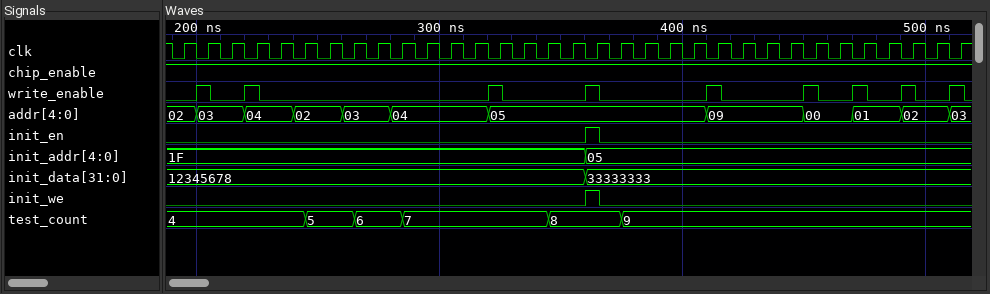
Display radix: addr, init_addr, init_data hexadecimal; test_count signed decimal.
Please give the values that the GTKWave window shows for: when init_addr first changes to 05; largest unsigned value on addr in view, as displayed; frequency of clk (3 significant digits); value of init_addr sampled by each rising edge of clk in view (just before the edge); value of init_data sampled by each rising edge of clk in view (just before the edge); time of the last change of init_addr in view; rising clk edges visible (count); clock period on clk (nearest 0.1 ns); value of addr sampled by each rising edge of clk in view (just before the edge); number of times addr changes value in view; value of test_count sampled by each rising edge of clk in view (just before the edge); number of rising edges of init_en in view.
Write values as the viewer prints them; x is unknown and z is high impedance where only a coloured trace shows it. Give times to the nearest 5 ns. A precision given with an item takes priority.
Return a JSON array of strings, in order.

["360 ns", "09", "100 MHz", "1F, 1F, 1F, 1F, 1F, 1F, 1F, 1F, 1F, 1F, 1F, 1F, 1F, 1F, 1F, 1F, 1F, 05, 05, 05, 05, 05, 05, 05, 05, 05, 05, 05, 05, 05, 05, 05, 05", "12345678, 12345678, 12345678, 12345678, 12345678, 12345678, 12345678, 12345678, 12345678, 12345678, 12345678, 12345678, 12345678, 12345678, 12345678, 12345678, 12345678, 33333333, 33333333, 33333333, 33333333, 33333333, 33333333, 33333333, 33333333, 33333333, 33333333, 33333333, 33333333, 33333333, 33333333, 33333333, 33333333", "360 ns", "33", "10 ns", "02, 03, 03, 04, 04, 02, 02, 03, 03, 04, 04, 04, 04, 05, 05, 05, 05, 05, 05, 05, 05, 05, 09, 09, 09, 09, 00, 00, 01, 01, 02, 02, 03", "11", "4, 4, 4, 4, 4, 4, 5, 5, 6, 6, 7, 7, 7, 7, 7, 7, 8, 8, 8, 9, 9, 9, 9, 9, 9, 9, 9, 9, 9, 9, 9, 9, 9", "1"]
